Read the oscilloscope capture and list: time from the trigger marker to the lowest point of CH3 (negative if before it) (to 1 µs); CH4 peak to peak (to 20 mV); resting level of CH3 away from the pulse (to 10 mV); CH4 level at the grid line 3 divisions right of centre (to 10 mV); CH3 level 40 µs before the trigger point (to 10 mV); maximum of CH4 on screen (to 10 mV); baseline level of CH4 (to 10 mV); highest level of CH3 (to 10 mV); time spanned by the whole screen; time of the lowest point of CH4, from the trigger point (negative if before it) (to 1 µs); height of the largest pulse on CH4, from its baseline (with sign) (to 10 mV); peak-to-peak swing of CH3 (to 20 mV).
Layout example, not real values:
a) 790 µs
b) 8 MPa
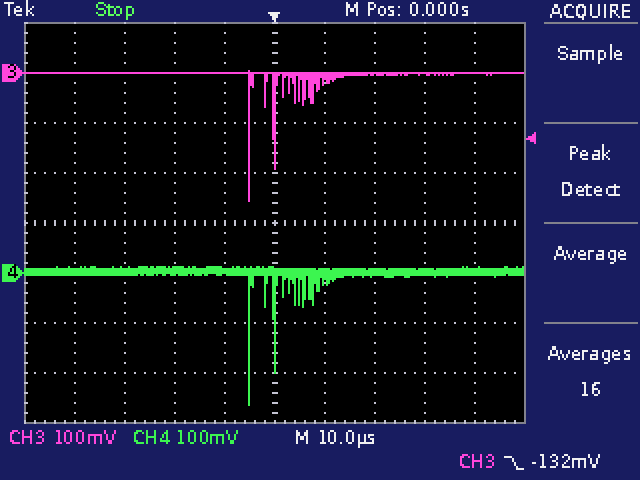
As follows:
a) -5 µs
b) 280 mV
c) 0 mV
d) 0 mV
e) 0 mV
f) 10 mV
g) 0 mV
h) 0 mV
i) 100 µs
j) -5 µs
k) -270 mV
l) 260 mV
